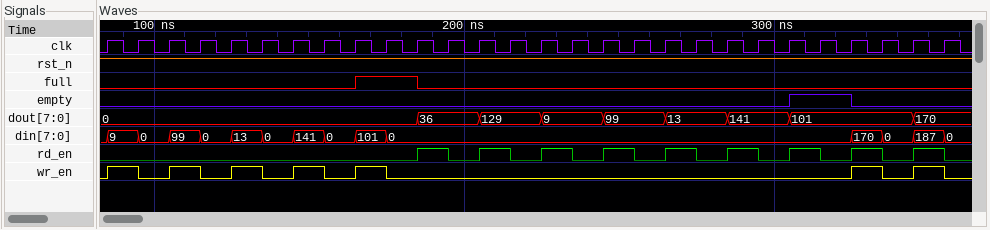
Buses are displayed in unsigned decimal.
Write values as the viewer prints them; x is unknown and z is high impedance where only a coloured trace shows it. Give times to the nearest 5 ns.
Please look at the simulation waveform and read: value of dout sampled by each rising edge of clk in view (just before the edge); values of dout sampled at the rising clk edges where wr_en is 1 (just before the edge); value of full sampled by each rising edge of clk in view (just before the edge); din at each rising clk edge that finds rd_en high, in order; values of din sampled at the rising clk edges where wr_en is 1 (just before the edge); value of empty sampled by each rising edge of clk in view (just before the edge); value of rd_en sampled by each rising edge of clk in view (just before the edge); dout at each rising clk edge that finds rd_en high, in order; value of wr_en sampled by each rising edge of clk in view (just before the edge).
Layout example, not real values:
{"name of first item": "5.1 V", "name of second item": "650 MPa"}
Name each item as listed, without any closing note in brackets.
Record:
{"value of dout sampled by each rising edge of clk in view": "0, 0, 0, 0, 0, 0, 0, 0, 0, 0, 0, 36, 36, 129, 129, 9, 9, 99, 99, 13, 13, 141, 141, 101, 101, 101, 101, 170", "values of dout sampled at the rising clk edges where wr_en is 1": "0, 0, 0, 0, 0, 101, 170", "value of full sampled by each rising edge of clk in view": "0 0 0 0 0 0 0 0 0 1 1 0 0 0 0 0 0 0 0 0 0 0 0 0 0 0 0 0", "din at each rising clk edge that finds rd_en high, in order": "0, 0, 0, 0, 0, 0, 0, 170, 187", "values of din sampled at the rising clk edges where wr_en is 1": "9, 99, 13, 141, 101, 170, 187", "value of empty sampled by each rising edge of clk in view": "0 0 0 0 0 0 0 0 0 0 0 0 0 0 0 0 0 0 0 0 0 0 0 1 1 0 0 0", "value of rd_en sampled by each rising edge of clk in view": "0 0 0 0 0 0 0 0 0 0 0 1 0 1 0 1 0 1 0 1 0 1 0 1 0 1 0 1", "dout at each rising clk edge that finds rd_en high, in order": "36, 129, 9, 99, 13, 141, 101, 101, 170", "value of wr_en sampled by each rising edge of clk in view": "0 1 0 1 0 1 0 1 0 1 0 0 0 0 0 0 0 0 0 0 0 0 0 0 0 1 0 1"}
